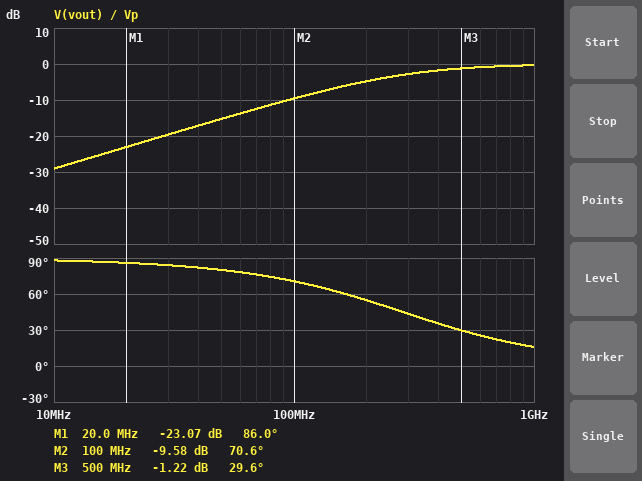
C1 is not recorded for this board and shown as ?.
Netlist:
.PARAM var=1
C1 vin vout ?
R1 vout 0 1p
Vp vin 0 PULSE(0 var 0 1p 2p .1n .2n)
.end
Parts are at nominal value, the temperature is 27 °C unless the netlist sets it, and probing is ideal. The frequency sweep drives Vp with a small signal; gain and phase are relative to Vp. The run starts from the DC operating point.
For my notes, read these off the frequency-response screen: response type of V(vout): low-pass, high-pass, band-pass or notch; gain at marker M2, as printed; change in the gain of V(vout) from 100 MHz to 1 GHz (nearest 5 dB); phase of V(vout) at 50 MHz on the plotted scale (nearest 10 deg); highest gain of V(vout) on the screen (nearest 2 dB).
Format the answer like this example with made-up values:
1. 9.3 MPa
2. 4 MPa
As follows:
1. high-pass
2. -9.58 dB
3. 10 dB
4. 80 deg
5. 0 dB
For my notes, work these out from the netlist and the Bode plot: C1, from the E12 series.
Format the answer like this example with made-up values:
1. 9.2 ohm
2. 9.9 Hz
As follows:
1. 560 F
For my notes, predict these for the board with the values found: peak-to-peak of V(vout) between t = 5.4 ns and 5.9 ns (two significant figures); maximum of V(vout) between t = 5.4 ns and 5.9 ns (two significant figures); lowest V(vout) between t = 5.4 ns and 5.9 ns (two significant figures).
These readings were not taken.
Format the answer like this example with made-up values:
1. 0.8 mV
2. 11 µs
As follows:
1. 1.1 V
2. 540 mV
3. -550 mV
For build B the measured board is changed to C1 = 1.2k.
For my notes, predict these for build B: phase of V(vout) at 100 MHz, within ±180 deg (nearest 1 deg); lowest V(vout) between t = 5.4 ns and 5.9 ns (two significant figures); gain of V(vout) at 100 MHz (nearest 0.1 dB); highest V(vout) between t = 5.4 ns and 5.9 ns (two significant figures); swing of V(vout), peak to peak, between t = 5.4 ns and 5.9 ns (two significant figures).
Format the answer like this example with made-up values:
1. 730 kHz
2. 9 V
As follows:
1. 53 deg
2. -520 mV
3. -4.4 dB
4. 520 mV
5. 1.0 V
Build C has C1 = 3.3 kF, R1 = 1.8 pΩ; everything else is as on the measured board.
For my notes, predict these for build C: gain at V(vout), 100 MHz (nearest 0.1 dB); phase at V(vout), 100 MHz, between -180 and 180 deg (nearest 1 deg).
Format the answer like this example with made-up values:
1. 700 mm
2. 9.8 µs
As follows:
1. -0.3 dB
2. 15 deg
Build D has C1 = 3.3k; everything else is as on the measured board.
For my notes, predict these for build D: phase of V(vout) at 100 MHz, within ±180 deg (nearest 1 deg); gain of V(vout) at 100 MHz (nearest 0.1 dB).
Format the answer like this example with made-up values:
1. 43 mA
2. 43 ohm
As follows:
1. 26 deg
2. -0.9 dB
